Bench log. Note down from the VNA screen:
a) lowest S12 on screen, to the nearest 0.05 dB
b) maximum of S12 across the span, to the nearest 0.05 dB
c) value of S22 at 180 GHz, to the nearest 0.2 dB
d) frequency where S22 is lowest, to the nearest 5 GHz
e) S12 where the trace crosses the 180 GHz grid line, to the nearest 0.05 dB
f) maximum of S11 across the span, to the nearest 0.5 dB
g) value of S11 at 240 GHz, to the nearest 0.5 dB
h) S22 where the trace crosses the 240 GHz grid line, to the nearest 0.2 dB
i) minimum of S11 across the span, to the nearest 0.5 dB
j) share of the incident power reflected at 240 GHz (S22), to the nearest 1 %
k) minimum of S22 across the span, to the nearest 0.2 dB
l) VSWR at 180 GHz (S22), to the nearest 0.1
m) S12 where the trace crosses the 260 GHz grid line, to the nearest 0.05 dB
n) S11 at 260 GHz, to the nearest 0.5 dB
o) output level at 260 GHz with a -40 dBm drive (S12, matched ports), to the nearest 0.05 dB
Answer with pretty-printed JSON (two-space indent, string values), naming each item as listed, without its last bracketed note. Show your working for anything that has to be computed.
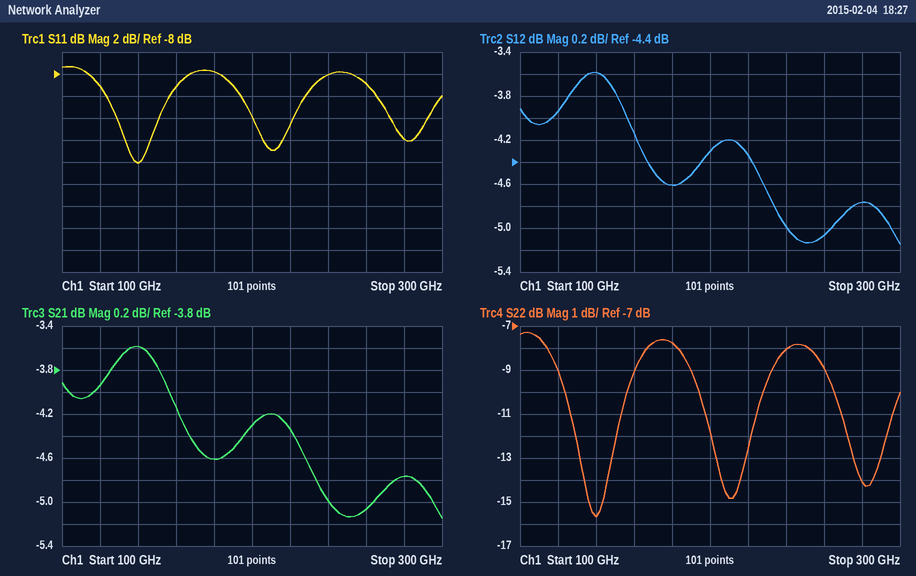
{
  "lowest S12 on screen, to the nearest 0.05 dB": "-5.15 dB",
  "maximum of S12 across the span, to the nearest 0.05 dB": "-3.60 dB",
  "value of S22 at 180 GHz, to the nearest 0.2 dB": "-7.8 dB",
  "frequency where S22 is lowest, to the nearest 5 GHz": "140 GHz",
  "S12 where the trace crosses the 180 GHz grid line, to the nearest 0.05 dB": "-4.60 dB",
  "maximum of S11 across the span, to the nearest 0.5 dB": "-7.5 dB",
  "value of S11 at 240 GHz, to the nearest 0.5 dB": "-8.0 dB",
  "S22 where the trace crosses the 240 GHz grid line, to the nearest 0.2 dB": "-8.0 dB",
  "minimum of S11 across the span, to the nearest 0.5 dB": "-16.0 dB",
  "share of the incident power reflected at 240 GHz (S22), to the nearest 1 %": "10^(-8/10) ≈ 16 %",
  "minimum of S22 across the span, to the nearest 0.2 dB": "-15.6 dB",
  "VSWR at 180 GHz (S22), to the nearest 0.1": "|Γ| = 10^(-7.8/20) = 0.4074; VSWR = (1 + 0.4074)/(1 − 0.4074) ≈ 2.4",
  "S12 where the trace crosses the 260 GHz grid line, to the nearest 0.05 dB": "-5.05 dB",
  "S11 at 260 GHz, to the nearest 0.5 dB": "-9.0 dB",
  "output level at 260 GHz with a -40 dBm drive (S12, matched ports), to the nearest 0.05 dB": "-40 dBm + (-5.05 dB) = -45.05 dBm"
}
